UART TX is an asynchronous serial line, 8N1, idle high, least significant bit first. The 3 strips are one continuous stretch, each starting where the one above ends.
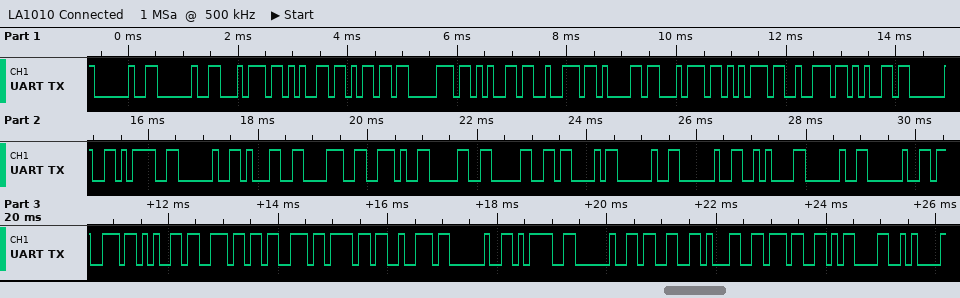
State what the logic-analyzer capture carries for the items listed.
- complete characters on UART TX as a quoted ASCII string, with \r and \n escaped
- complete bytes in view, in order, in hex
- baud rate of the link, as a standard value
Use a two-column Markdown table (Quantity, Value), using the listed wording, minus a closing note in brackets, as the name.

| Quantity | Value |
|---|---|
| complete characters on UART TX as a quoted ASCII string, with \r and \n escaped | "  temperature = 18.00C  \n  sensor = 317\r\n" |
| complete bytes in view, in order, in hex | 20 20 74 65 6D 70 65 72 61 74 75 72 65 20 3D 20 31 38 2E 30 30 43 20 20 0A 20 20 73 65 6E 73 6F 72 20 3D 20 33 31 37 0D 0A |
| baud rate of the link, as a standard value | 9600 baud |
